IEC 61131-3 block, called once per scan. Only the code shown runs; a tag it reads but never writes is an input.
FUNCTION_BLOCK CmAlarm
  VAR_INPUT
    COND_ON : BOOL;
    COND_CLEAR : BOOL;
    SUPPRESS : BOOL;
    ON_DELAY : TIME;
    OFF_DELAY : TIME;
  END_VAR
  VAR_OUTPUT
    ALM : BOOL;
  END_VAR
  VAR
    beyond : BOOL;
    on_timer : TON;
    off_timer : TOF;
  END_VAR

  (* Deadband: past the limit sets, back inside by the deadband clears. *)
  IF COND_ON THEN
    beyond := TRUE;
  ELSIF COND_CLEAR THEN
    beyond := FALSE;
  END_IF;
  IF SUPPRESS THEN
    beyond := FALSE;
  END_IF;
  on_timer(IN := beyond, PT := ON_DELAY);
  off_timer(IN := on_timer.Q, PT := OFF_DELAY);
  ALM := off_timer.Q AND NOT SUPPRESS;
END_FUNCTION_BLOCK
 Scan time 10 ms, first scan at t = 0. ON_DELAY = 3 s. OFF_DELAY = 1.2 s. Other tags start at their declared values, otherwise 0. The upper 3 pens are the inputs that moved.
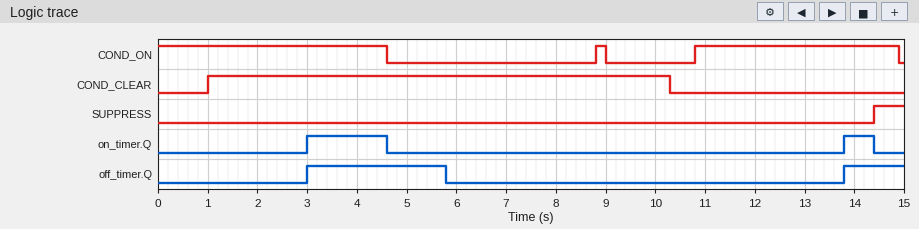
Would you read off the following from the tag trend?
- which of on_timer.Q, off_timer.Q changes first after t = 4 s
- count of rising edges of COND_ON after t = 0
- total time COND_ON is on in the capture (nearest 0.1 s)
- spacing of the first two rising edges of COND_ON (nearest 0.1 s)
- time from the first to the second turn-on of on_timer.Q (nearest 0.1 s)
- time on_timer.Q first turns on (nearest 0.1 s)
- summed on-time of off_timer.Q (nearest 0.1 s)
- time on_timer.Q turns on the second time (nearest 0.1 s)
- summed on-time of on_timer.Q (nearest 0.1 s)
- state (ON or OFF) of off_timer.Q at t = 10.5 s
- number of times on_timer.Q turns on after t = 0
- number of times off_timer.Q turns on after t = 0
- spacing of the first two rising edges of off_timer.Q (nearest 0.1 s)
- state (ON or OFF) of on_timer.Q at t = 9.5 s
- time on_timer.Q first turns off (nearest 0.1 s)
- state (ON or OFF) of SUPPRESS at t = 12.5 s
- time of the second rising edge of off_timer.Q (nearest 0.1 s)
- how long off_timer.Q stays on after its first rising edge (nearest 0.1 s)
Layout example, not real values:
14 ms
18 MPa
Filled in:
on_timer.Q
2
8.9 s
2.0 s
10.8 s
3.0 s
4.0 s
13.8 s
2.2 s
OFF
2
2
10.8 s
OFF
4.6 s
OFF
13.8 s
2.8 s
